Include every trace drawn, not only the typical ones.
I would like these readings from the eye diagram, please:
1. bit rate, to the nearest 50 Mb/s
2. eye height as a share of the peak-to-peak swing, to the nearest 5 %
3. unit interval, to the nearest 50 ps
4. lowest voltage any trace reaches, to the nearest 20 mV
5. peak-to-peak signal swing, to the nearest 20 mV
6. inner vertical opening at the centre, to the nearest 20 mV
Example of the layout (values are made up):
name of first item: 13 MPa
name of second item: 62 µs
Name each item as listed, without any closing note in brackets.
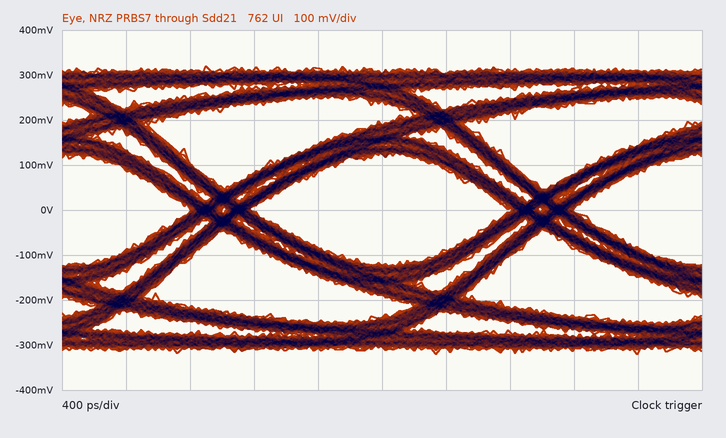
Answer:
bit rate, to the nearest 50 Mb/s: 500 Mb/s
eye height as a share of the peak-to-peak swing, to the nearest 5 %: 40 %
unit interval, to the nearest 50 ps: 2.00 ns
lowest voltage any trace reaches, to the nearest 20 mV: -320 mV
peak-to-peak signal swing, to the nearest 20 mV: 640 mV
inner vertical opening at the centre, to the nearest 20 mV: 240 mV
